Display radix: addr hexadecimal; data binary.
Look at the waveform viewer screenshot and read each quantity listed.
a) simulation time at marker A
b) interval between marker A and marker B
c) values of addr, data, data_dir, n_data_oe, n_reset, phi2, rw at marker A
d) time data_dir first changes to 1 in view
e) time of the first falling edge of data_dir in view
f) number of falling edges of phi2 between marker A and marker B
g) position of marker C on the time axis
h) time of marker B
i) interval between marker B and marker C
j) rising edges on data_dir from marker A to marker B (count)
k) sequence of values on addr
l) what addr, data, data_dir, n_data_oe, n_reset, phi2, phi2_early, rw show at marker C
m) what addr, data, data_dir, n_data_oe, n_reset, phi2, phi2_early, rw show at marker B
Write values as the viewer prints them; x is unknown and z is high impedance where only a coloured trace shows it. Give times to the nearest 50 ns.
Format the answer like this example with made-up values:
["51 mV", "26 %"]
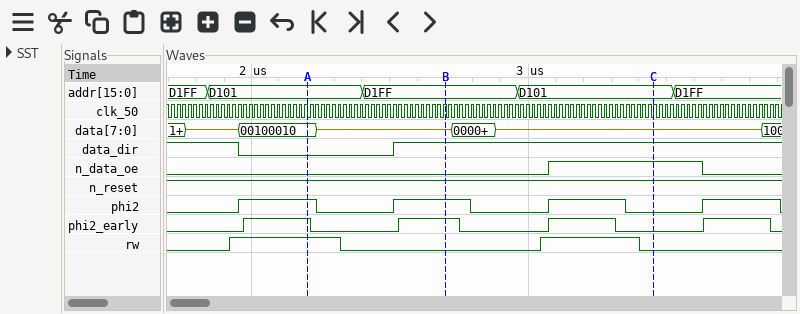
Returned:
["2200 ns", "500 ns", "addr=D101, data=00100010, data_dir=0, n_data_oe=0, n_reset=1, phi2=1, rw=1", "2500 ns", "1950 ns", "1", "3450 ns", "2700 ns", "750 ns", "1", "D1FF, D101, D1FF, D101, D1FF", "addr=D101, data=z, data_dir=1, n_data_oe=1, n_reset=1, phi2=0, phi2_early=0, rw=0", "addr=D1FF, data=z, data_dir=1, n_data_oe=0, n_reset=1, phi2=1, phi2_early=1, rw=0"]
